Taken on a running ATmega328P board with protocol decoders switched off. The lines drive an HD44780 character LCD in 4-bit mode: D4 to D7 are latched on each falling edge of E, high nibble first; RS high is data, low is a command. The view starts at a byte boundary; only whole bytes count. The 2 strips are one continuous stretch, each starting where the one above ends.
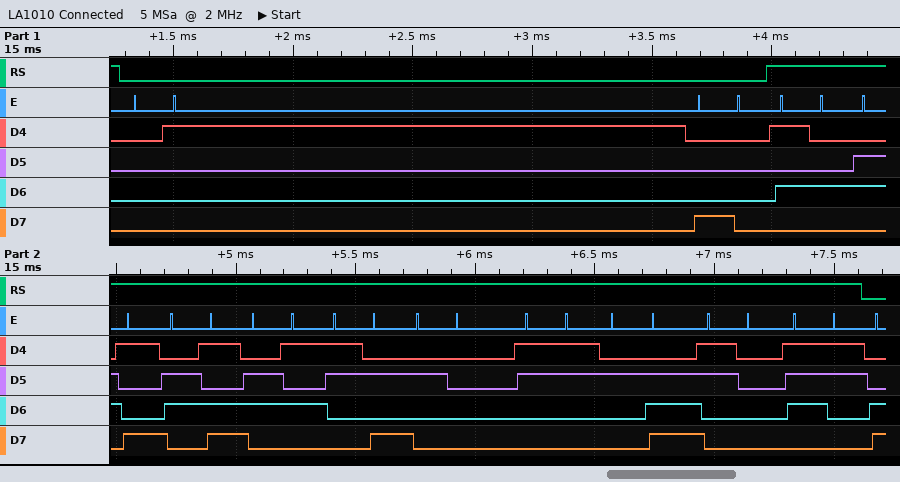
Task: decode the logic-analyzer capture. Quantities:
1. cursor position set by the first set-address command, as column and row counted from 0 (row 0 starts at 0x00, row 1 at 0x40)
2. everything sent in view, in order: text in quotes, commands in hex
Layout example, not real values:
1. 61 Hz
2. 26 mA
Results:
1. column 0, row 0
2. 0x01 0x80 "Time: 3.0s"
